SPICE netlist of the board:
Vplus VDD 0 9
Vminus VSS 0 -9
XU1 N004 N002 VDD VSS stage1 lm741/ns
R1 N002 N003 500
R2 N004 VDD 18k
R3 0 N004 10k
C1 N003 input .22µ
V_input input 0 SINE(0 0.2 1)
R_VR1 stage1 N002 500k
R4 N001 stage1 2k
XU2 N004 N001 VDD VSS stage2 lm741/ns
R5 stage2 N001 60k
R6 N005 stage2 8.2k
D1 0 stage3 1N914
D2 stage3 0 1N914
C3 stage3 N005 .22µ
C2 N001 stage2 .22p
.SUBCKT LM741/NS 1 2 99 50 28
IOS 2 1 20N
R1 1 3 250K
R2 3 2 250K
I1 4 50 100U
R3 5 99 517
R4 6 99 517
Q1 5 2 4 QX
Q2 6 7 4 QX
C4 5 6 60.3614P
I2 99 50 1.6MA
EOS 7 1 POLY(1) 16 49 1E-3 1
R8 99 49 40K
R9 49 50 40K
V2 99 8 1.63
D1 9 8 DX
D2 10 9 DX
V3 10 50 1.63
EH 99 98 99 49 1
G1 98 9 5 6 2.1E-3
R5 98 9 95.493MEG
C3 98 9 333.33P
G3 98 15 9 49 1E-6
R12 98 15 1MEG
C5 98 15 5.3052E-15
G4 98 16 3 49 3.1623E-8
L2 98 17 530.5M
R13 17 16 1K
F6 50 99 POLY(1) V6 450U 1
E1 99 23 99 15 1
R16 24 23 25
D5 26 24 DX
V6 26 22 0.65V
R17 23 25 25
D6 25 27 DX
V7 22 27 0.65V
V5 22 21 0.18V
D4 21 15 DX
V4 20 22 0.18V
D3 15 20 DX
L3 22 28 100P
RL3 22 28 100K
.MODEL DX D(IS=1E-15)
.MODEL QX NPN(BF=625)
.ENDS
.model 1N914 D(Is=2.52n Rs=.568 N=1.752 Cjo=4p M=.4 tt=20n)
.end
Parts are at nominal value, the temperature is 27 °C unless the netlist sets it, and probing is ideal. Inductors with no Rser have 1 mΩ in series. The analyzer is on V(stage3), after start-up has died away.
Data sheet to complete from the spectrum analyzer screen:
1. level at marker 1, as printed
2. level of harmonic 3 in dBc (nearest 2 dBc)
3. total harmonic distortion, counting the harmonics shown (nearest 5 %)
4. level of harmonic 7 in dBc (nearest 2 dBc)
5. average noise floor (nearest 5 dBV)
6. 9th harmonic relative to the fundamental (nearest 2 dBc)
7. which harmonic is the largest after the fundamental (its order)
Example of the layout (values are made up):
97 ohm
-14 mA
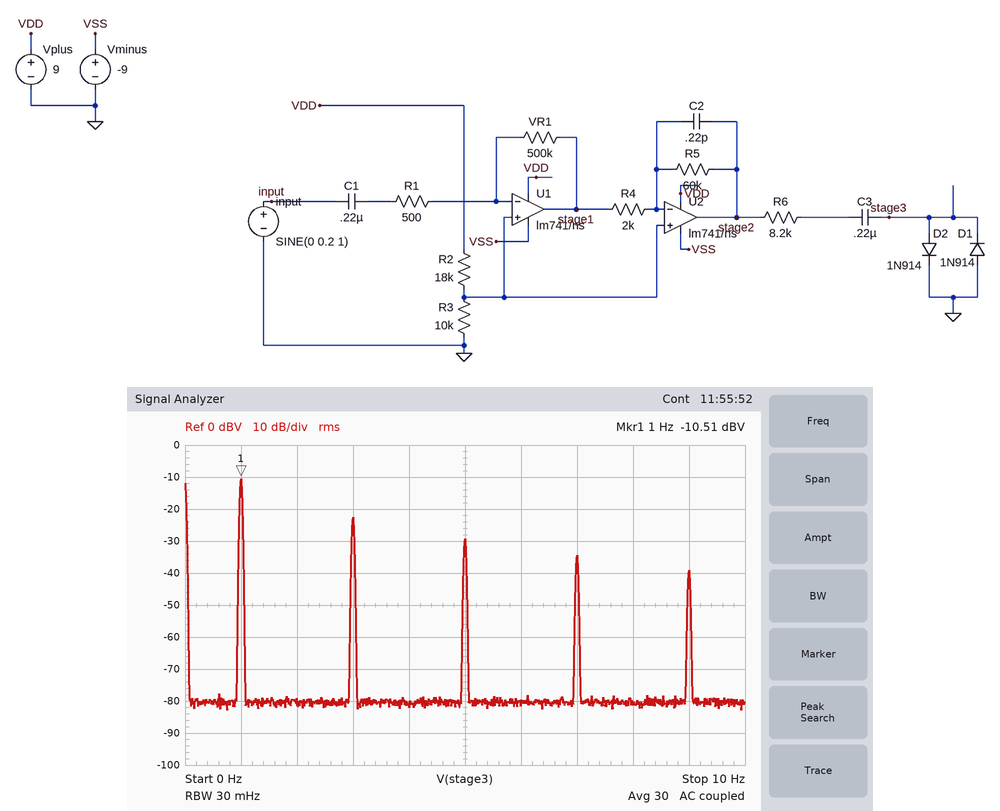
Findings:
-10.51 dBV
-12 dBc
30 %
-24 dBc
-80 dBV
-28 dBc
3
